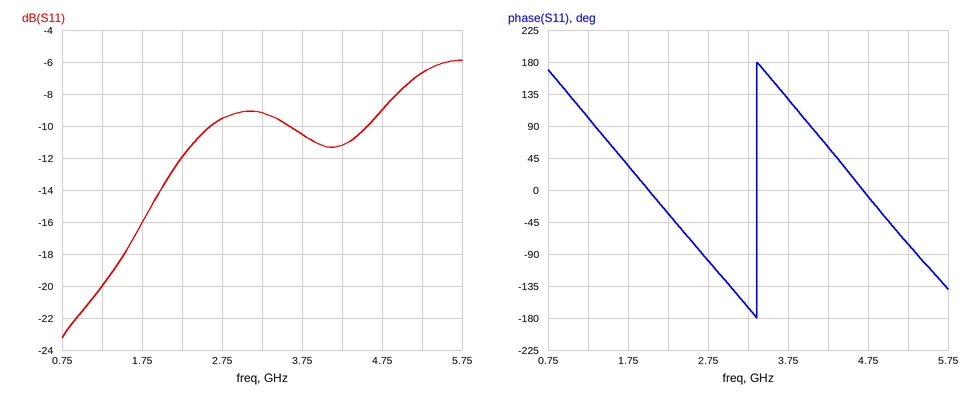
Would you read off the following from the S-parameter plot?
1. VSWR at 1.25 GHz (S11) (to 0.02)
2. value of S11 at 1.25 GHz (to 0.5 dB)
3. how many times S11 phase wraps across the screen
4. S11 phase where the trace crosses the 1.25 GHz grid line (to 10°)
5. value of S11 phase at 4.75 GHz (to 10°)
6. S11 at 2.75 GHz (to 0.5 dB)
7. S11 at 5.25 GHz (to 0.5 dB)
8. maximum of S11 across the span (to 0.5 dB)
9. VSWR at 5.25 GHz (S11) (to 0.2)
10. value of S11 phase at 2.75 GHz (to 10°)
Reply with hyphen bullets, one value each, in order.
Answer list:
- 1.22
- -20.0 dB
- 1
- 100°
- -10°
- -9.5 dB
- -6.5 dB
- -6.0 dB
- 2.8
- -100°
